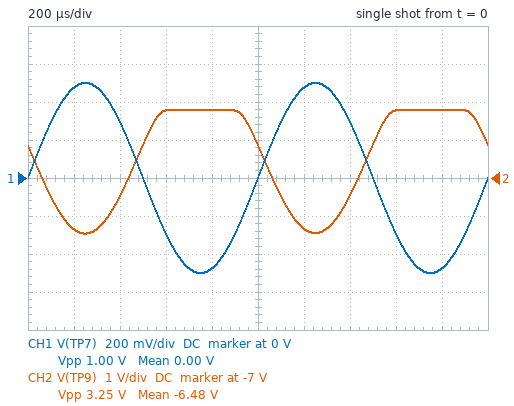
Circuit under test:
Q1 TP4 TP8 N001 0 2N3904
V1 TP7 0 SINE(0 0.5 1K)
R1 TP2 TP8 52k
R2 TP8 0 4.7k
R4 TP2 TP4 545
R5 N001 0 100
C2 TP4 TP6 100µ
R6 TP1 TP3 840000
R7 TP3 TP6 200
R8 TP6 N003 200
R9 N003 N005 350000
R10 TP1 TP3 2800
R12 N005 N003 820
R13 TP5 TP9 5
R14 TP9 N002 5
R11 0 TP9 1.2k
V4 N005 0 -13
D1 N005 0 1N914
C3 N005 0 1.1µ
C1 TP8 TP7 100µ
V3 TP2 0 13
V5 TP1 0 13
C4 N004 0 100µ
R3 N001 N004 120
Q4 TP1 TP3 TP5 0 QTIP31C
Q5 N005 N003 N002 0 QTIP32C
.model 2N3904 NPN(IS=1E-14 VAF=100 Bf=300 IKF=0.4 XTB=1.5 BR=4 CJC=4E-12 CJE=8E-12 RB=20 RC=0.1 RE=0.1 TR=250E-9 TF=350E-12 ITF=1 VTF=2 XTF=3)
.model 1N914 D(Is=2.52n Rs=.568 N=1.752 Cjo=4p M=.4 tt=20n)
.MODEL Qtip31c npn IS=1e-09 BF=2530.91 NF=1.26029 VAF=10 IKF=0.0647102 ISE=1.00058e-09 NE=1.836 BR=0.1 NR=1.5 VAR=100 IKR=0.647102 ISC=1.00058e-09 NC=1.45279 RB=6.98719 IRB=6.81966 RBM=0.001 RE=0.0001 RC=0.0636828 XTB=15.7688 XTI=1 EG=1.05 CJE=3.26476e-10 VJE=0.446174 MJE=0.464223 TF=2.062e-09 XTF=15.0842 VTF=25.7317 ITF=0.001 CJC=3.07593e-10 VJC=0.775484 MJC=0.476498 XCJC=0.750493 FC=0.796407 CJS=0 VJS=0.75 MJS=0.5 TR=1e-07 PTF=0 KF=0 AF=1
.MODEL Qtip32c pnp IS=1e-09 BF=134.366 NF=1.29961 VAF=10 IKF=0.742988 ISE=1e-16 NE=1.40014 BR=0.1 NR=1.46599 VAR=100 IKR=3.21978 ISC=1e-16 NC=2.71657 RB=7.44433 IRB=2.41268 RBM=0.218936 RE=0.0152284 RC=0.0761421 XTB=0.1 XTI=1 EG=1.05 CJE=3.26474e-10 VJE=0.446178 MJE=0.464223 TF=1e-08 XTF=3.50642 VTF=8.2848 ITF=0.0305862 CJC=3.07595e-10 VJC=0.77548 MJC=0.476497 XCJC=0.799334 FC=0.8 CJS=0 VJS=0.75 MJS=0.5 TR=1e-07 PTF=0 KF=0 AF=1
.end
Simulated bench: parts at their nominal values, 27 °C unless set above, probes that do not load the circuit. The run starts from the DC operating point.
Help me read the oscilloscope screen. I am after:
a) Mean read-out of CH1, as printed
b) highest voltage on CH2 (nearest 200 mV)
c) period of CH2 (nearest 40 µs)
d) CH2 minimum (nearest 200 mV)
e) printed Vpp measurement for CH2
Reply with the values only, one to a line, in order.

0.00 V
-5.2 V
1.00 ms
-8.4 V
3.25 V
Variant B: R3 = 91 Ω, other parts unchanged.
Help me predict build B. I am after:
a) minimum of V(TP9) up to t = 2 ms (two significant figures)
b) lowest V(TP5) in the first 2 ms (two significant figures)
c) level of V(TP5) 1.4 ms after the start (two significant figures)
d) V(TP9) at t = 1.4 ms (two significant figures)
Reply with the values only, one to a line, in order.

-8.8 V
-8.3 V
-7.1 V
-7.6 V
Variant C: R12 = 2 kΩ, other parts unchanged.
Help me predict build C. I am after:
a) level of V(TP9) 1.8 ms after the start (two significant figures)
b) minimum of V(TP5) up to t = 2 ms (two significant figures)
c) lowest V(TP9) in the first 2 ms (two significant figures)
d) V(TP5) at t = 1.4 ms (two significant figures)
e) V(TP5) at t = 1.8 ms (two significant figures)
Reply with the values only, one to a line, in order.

-700 mV
-4.5 V
-4.8 V
-3.2 V
-310 mV
